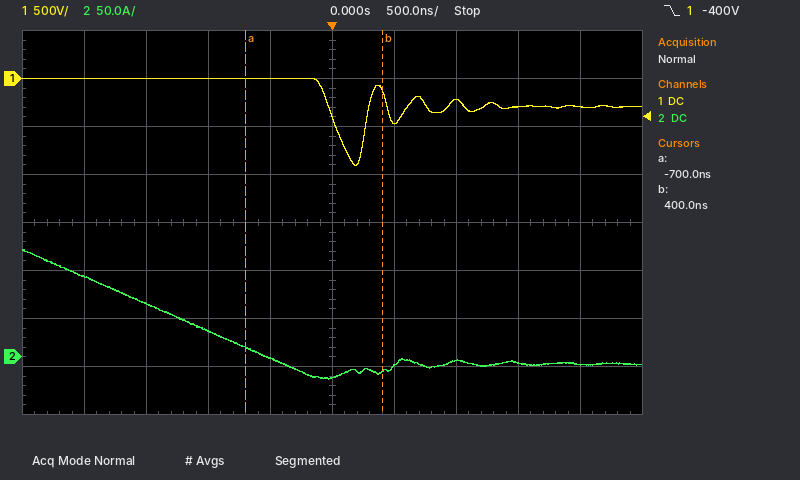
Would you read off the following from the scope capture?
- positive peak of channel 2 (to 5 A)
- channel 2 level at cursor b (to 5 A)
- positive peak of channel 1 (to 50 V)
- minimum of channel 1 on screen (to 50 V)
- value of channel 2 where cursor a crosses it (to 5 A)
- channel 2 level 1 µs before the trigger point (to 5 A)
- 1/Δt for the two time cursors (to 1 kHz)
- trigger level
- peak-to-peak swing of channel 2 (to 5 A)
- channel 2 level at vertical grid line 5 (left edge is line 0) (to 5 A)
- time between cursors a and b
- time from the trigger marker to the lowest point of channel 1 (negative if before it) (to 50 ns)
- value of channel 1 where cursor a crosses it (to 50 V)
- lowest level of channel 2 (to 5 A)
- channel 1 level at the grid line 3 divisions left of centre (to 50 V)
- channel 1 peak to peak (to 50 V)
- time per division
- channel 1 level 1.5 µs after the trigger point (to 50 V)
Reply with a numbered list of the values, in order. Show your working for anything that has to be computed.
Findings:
1. 110 A
2. -15 A
3. 0 V
4. -900 V
5. 10 A
6. 25 A
7. 1 / 1.10 µs ≈ 909 kHz
8. -400 V
9. 110 A − (-25 A) = 135 A
10. -20 A
11. 400 ns − (-700 ns) = 1.10 µs
12. +200 ns
13. 0 V
14. -25 A
15. 0 V
16. 0 V − (-900 V) = 900 V
17. 500 ns
18. -300 V
